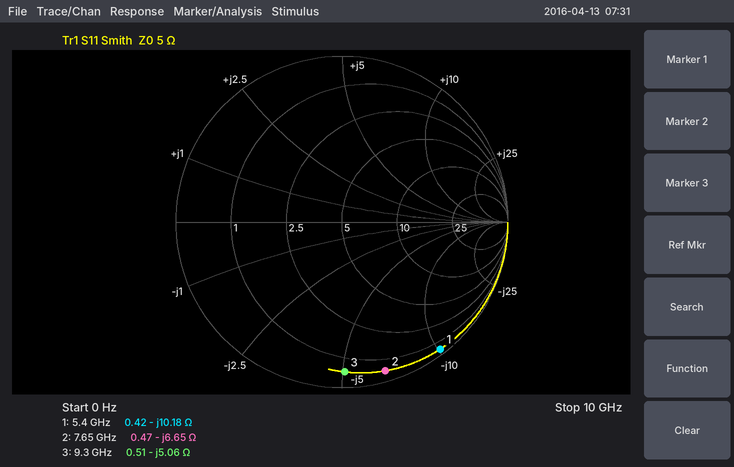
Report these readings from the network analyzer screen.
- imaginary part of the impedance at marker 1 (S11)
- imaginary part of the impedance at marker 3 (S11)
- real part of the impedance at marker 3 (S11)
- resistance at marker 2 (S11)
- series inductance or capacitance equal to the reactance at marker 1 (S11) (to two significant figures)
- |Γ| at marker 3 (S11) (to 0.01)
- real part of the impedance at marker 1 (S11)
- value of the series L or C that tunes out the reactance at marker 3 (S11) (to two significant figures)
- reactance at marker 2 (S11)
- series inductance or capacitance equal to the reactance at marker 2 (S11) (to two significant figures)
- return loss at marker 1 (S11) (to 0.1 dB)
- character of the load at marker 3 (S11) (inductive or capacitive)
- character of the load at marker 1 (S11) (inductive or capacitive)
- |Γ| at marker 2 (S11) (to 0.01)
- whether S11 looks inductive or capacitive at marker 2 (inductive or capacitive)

-10.18 Ω
-5.06 Ω
0.51 Ω
0.47 Ω
2.9 pF
0.90
0.42 Ω
87 pH
-6.65 Ω
3.1 pF
0.3 dB
capacitive
capacitive
0.93
capacitive
